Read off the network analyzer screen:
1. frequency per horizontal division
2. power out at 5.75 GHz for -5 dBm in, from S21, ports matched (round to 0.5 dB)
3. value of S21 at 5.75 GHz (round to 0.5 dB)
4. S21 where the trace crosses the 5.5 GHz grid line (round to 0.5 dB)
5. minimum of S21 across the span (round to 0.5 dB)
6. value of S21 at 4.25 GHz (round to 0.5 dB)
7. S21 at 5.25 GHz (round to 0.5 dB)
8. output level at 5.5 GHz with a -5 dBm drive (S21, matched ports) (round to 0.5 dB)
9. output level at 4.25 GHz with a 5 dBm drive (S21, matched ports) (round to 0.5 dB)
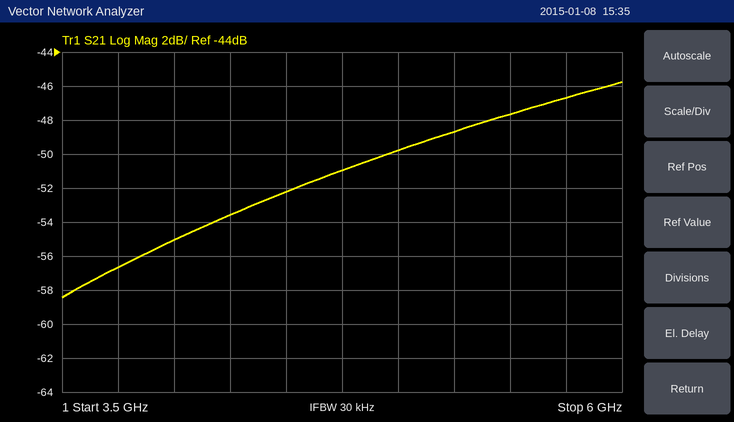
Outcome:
250 MHz
-51.5 dBm
-46.5 dB
-47.5 dB
-58.5 dB
-53.5 dB
-48.5 dB
-52.5 dBm
-48.5 dBm
